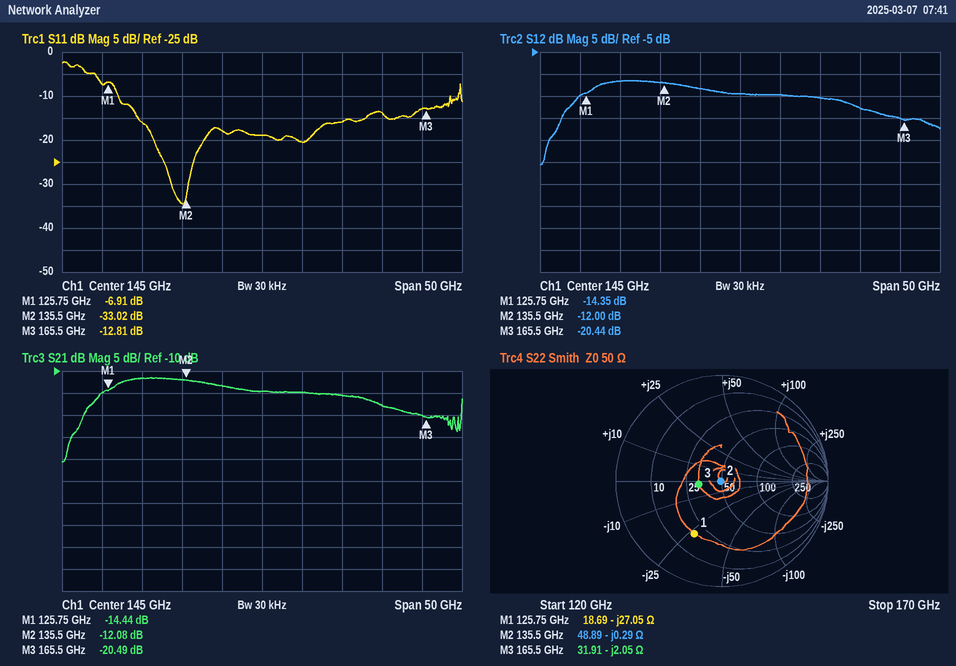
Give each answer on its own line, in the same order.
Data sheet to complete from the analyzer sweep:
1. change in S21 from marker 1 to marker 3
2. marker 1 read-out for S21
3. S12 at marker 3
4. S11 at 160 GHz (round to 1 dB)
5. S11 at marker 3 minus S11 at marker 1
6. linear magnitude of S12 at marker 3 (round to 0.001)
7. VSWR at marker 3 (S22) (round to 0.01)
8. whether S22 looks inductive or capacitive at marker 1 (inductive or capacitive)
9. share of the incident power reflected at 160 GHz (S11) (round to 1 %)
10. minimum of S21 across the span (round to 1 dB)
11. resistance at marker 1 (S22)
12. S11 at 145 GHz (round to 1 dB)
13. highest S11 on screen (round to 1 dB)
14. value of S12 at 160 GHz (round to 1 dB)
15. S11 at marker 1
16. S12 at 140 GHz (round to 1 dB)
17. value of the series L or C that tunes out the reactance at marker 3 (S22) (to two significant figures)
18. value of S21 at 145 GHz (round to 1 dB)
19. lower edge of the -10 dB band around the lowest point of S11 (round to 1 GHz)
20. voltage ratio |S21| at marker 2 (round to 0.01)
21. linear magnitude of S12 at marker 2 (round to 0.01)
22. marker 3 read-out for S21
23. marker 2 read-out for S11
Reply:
-6.05 dB
-14.44 dB
-20.44 dB
-14 dB
-5.90 dB
0.095
1.57
capacitive
4 %
-31 dB
18.69 Ω
-19 dB
-2 dB
-18 dB
-6.91 dB
-13 dB
2.0 pH
-15 dB
127 GHz
0.25
0.25
-20.49 dB
-33.02 dB
